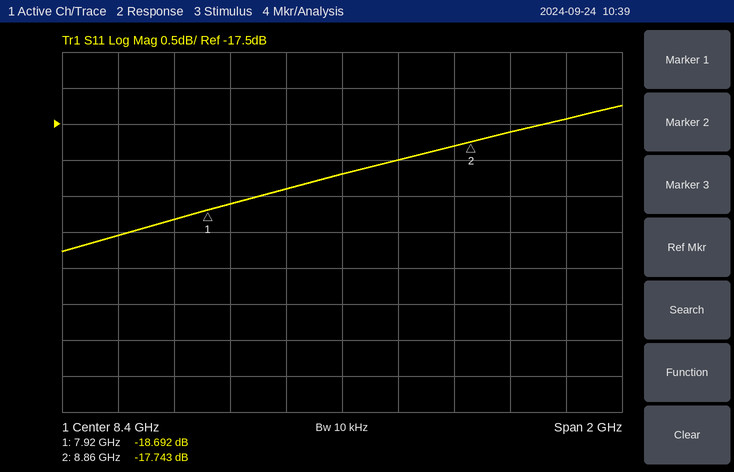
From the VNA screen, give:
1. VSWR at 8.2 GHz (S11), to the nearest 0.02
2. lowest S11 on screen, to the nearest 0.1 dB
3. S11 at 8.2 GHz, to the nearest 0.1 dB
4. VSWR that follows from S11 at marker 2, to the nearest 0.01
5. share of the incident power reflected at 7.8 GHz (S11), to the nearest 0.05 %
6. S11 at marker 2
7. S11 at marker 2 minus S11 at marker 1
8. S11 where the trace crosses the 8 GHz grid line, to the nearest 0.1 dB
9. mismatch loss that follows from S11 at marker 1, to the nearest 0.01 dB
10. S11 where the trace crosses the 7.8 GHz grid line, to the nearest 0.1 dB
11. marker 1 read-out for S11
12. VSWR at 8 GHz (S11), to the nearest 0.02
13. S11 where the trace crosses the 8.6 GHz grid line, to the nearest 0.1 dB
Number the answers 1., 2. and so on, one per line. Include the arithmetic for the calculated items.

1. |Γ| = 10^(-18.4/20) = 0.1202; VSWR = (1 + 0.1202)/(1 − 0.1202) ≈ 1.27, so 1.28 to the nearest 0.02
2. -19.3 dB
3. -18.4 dB
4. (1 + 0.1297)/(1 − 0.1297) ≈ 1.30
5. 10^(-18.8/10) ≈ 1.32 %, so 1.30 % to the nearest 0.05 %
6. -17.743 dB
7. -17.743 − (-18.692) = 0.949 dB
8. -18.6 dB
9. −10 log10(1 − 10^(-18.692/10)) ≈ 0.06 dB
10. -18.8 dB
11. -18.692 dB
12. |Γ| = 10^(-18.6/20) = 0.1175; VSWR = (1 + 0.1175)/(1 − 0.1175) ≈ 1.27, so 1.26 to the nearest 0.02
13. -18.0 dB
